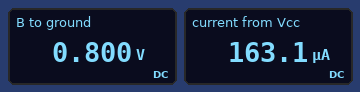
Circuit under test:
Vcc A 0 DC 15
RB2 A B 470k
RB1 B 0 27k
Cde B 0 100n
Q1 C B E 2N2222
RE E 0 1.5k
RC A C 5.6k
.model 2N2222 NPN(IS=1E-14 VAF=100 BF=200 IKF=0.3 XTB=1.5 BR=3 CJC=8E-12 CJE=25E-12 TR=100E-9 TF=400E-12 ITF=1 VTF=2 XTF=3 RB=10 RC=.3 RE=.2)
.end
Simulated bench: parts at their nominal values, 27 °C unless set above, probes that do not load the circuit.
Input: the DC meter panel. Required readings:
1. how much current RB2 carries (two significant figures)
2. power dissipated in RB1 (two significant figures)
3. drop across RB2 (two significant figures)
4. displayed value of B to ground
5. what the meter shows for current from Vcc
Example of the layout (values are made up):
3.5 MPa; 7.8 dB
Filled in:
30 µA; 24 µW; 14 V; 0.800 V; 163.1 µA
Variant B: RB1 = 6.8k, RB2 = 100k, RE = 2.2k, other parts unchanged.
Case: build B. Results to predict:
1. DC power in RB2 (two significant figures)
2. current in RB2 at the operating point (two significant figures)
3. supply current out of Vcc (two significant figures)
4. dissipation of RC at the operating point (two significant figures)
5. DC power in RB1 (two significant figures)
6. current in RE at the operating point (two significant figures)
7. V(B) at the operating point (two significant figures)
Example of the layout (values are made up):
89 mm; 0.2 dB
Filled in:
2.0 mW; 140 µA; 300 µA; 140 µW; 130 µW; 160 µA; 950 mV
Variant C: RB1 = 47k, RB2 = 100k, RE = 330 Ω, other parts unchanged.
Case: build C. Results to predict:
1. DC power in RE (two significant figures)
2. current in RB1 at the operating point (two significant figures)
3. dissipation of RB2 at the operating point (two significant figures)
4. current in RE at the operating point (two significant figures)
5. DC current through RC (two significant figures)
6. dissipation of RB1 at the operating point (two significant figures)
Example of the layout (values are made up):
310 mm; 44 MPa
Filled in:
2.3 mW; 33 µA; 1.8 mW; 2.6 mA; 2.5 mA; 51 µW
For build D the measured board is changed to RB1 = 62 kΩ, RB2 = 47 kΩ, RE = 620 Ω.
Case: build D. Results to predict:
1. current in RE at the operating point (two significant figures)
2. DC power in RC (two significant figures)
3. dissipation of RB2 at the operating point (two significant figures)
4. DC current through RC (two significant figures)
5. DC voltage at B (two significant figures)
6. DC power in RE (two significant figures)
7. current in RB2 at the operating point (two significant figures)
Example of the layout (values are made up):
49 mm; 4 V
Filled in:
2.6 mA; 32 mW; 3.4 mW; 2.4 mA; 2.3 V; 4.2 mW; 270 µA
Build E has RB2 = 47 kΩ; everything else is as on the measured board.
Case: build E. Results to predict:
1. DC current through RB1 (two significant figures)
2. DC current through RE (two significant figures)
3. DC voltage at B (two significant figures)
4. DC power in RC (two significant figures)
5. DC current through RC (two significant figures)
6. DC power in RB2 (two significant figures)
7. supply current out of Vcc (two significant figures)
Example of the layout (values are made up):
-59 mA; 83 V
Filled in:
150 µA; 2.2 mA; 3.9 V; 24 mW; 2.1 mA; 2.6 mW; 2.3 mA
